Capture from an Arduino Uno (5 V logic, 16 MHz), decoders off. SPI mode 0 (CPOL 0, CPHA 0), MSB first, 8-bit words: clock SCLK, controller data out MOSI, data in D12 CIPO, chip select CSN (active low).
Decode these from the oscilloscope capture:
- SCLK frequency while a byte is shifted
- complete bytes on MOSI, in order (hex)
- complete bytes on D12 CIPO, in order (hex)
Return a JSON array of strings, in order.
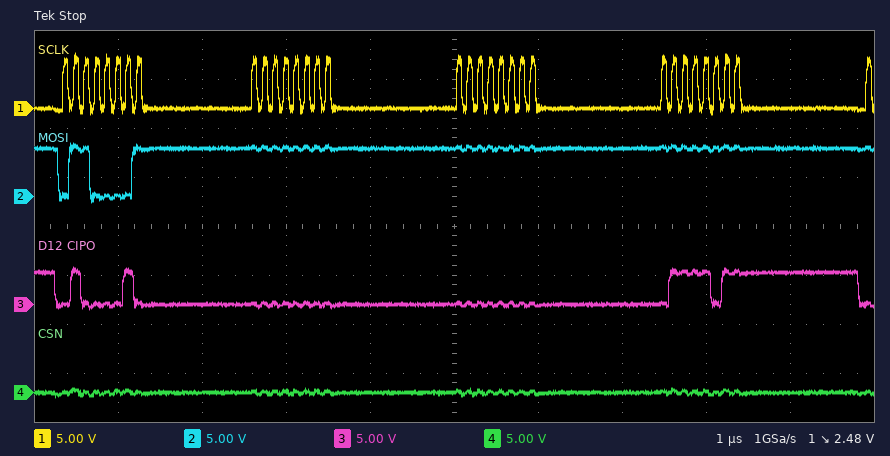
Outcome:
["8 MHz", "61 FF FF FF", "42 00 00 7B"]
